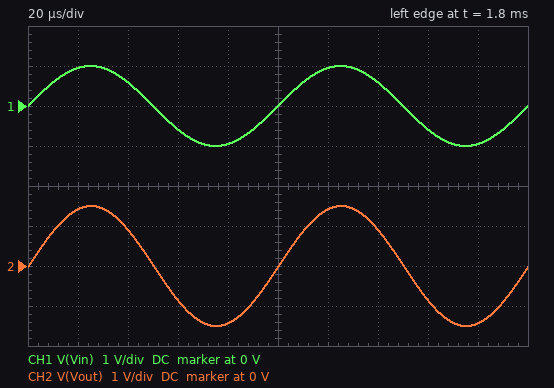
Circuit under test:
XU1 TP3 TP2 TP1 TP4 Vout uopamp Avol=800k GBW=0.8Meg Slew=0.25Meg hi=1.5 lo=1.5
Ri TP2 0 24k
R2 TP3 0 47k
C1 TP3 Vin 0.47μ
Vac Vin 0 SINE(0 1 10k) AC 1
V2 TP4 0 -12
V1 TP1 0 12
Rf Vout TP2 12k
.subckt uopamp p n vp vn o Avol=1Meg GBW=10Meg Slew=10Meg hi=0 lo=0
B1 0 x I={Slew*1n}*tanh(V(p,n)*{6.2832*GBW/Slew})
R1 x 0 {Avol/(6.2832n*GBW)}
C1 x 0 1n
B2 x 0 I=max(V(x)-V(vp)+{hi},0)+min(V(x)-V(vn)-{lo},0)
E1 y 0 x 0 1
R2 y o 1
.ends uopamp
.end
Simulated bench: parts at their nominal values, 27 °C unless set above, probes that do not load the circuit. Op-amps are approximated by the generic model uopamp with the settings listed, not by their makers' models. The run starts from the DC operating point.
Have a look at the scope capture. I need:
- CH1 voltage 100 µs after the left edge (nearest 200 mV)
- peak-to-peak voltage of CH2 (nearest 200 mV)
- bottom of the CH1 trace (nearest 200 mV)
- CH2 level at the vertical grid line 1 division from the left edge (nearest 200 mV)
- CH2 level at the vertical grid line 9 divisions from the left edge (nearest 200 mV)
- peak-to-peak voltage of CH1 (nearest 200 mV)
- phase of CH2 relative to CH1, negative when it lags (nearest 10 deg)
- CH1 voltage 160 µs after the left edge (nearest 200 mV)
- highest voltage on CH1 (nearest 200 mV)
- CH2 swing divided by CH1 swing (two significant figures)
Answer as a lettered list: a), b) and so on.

a) 0 V
b) 3.0 V
c) -1.0 V
d) 1.4 V
e) -1.4 V
f) 2.0 V
g) 0 deg
h) -600 mV
i) 1.0 V
j) 1.5
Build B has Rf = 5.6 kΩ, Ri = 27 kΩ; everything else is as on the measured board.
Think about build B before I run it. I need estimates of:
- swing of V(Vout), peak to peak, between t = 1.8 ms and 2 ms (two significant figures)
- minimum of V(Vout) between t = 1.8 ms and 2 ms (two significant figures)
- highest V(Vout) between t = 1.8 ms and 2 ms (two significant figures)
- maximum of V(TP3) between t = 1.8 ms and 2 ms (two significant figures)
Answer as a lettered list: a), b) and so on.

a) 2.4 V
b) -1.2 V
c) 1.2 V
d) 1.0 V
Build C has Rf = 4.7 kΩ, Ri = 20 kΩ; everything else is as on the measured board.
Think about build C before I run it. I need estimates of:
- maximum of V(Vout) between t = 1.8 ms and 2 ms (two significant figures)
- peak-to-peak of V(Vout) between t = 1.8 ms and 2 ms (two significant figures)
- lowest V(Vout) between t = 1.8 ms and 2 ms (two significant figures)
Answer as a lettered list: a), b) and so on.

a) 1.2 V
b) 2.5 V
c) -1.2 V
